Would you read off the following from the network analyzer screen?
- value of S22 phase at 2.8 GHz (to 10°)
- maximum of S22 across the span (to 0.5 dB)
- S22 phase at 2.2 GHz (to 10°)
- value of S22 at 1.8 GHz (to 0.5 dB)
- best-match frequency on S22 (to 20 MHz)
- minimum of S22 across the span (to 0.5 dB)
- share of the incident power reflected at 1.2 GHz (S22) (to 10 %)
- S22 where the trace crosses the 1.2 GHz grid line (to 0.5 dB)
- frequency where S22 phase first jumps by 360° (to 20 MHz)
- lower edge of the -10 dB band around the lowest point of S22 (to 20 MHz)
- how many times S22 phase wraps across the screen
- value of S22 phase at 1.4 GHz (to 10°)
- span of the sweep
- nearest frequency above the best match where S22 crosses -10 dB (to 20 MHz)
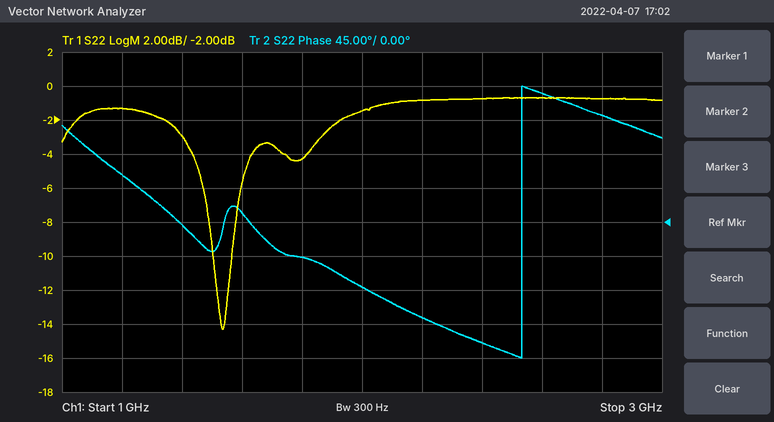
140°
-0.5 dB
-130°
-4.5 dB
1.54 GHz
-14.5 dB
70 %
-1.5 dB
2.54 GHz
1.50 GHz
1
0°
2 GHz
1.56 GHz
